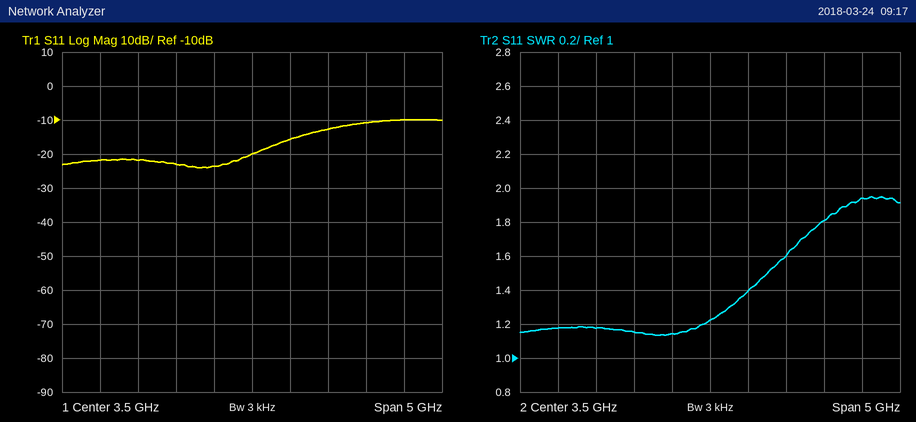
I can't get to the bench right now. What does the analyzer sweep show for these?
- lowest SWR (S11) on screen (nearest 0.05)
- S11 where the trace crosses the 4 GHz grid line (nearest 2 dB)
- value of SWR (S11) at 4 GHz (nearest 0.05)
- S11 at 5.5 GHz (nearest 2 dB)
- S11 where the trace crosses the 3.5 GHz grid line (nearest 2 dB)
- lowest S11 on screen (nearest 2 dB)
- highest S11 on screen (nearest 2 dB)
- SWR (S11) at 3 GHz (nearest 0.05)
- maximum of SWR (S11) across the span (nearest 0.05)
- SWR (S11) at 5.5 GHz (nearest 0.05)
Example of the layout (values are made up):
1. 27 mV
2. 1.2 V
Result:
1. 1.15
2. -16 dB
3. 1.40
4. -10 dB
5. -20 dB
6. -24 dB
7. -10 dB
8. 1.15
9. 1.95
10. 1.95
